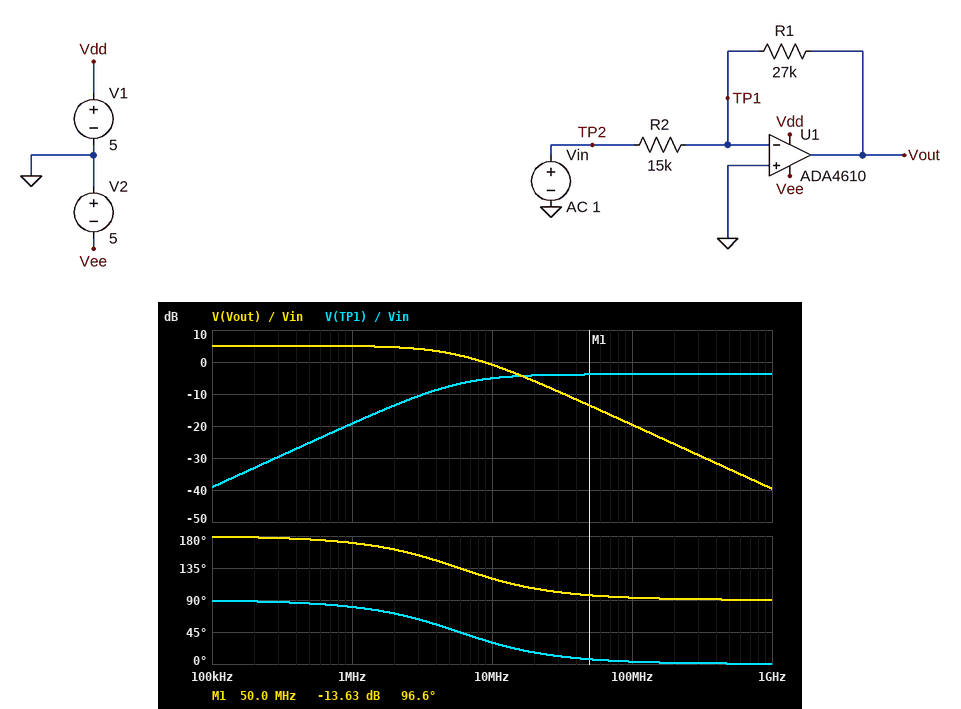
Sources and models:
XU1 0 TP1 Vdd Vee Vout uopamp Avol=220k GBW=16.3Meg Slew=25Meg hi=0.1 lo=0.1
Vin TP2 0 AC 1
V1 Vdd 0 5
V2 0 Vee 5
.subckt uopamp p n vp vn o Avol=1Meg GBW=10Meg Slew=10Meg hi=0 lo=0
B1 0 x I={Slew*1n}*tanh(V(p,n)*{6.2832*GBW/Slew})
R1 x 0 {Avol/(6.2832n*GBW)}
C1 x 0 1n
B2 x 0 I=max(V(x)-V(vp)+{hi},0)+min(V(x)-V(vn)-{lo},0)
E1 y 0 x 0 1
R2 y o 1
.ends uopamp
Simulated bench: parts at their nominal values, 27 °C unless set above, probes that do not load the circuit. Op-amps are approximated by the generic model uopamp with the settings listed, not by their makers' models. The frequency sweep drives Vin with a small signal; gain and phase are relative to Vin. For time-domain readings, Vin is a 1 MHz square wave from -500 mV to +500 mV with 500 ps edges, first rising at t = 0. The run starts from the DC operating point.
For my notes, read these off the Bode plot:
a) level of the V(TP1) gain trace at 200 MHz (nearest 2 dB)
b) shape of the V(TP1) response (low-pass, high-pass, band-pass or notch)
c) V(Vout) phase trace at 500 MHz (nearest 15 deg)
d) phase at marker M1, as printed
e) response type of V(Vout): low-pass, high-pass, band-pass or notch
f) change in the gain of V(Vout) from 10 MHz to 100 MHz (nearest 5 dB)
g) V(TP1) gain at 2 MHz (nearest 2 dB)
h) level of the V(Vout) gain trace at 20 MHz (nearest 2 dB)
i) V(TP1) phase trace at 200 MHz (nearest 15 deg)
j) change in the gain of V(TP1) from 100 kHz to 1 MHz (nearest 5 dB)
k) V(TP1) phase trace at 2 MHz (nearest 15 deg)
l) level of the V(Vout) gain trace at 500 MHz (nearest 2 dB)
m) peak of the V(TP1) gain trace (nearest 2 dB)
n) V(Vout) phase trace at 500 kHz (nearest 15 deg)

-4 dB
high-pass
90 deg
96.6 deg
low-pass
-20 dB
-14 dB
-6 dB
0 deg
20 dB
75 deg
-34 dB
-4 dB
180 deg
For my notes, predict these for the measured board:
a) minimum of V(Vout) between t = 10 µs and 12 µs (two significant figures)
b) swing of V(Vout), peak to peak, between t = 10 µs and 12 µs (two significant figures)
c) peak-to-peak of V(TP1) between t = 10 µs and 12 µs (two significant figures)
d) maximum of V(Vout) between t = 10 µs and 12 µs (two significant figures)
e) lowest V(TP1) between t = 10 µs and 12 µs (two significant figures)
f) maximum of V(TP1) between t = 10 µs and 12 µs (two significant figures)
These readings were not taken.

-900 mV
1.8 V
1.3 V
900 mV
-640 mV
640 mV
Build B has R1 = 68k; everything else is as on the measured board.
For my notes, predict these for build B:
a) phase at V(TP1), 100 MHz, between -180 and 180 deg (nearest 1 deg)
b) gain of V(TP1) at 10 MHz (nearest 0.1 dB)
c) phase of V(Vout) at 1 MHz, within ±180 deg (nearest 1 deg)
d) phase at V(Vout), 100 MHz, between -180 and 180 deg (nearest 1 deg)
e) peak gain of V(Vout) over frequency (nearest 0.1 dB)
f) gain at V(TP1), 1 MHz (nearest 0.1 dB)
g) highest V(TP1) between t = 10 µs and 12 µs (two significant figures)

2 deg
-2.1 dB
161 deg
92 deg
13.1 dB
-11.6 dB
820 mV
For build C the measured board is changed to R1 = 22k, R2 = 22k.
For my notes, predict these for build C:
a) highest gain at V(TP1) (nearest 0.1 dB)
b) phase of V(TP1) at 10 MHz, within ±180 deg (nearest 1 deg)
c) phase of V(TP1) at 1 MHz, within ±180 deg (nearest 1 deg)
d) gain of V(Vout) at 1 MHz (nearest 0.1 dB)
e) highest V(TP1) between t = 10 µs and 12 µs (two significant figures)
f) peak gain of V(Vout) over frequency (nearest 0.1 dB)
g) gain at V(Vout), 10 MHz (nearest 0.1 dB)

-6.0 dB
39 deg
83 deg
-0.1 dB
500 mV
0 dB
-4.0 dB
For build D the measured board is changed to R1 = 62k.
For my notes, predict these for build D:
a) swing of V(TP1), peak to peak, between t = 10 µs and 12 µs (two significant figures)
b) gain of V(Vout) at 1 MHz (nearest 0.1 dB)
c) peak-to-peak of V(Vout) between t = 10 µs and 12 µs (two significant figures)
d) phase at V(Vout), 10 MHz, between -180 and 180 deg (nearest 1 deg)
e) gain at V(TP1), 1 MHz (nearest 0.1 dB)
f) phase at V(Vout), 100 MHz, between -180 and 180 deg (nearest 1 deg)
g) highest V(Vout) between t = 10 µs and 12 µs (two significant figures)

1.6 V
11.9 dB
4.1 V
108 deg
-12.3 dB
92 deg
2.1 V
